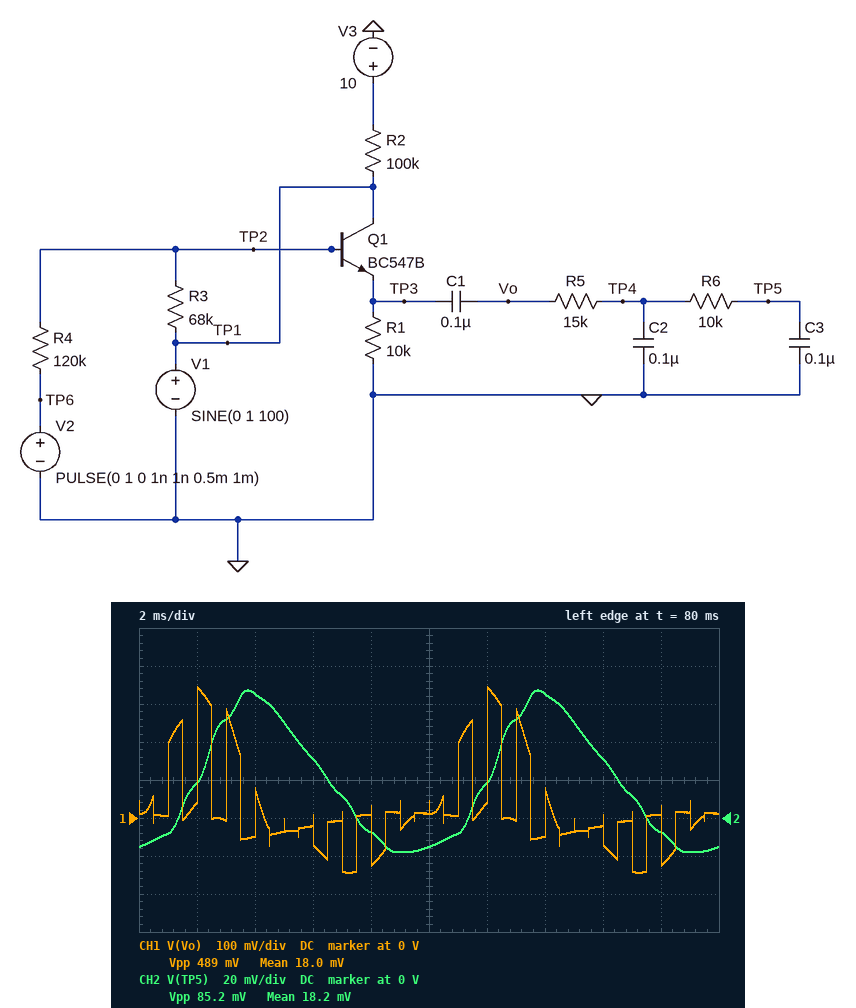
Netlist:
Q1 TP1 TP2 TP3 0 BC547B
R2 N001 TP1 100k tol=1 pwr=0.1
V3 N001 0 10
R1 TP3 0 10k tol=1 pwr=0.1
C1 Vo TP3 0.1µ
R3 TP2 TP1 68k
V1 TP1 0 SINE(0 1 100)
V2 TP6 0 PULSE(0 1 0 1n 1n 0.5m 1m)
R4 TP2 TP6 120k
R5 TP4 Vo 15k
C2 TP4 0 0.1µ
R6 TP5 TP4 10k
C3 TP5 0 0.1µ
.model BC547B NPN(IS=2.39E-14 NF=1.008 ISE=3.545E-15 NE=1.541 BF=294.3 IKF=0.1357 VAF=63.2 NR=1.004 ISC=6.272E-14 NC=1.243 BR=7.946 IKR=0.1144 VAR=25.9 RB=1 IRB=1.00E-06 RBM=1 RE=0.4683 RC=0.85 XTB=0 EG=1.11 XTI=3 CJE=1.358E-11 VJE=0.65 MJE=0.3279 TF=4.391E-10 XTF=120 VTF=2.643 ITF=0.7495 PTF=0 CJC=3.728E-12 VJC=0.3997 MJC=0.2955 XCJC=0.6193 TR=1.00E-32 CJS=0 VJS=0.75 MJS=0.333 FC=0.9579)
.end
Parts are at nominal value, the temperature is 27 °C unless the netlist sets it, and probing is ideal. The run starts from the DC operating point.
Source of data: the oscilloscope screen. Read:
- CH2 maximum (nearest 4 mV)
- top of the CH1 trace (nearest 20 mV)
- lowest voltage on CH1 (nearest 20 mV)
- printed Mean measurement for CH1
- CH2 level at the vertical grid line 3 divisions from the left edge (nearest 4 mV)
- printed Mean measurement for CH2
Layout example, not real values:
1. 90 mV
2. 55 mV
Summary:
1. 68 mV
2. 340 mV
3. -140 mV
4. 18.0 mV
5. 32 mV
6. 18.2 mV
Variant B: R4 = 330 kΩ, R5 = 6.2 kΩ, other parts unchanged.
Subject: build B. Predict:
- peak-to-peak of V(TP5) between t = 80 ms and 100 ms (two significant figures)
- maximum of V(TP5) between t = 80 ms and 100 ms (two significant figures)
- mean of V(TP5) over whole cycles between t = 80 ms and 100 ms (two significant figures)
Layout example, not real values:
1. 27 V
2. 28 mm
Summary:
1. 96 mV
2. 97 mV
3. 31 mV
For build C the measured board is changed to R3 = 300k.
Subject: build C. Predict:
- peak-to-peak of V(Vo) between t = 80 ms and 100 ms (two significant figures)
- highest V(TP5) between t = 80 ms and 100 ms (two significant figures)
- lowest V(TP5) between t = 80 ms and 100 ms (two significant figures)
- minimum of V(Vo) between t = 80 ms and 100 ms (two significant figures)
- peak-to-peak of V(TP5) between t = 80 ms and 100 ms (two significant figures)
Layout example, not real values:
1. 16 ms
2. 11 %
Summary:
1. 690 mV
2. 66 mV
3. -73 mV
4. -330 mV
5. 140 mV
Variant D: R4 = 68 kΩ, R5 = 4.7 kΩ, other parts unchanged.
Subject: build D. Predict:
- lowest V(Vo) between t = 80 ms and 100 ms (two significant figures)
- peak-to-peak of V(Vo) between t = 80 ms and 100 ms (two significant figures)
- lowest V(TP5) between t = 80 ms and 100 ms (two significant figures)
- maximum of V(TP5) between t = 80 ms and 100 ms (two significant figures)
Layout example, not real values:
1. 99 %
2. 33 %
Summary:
1. -280 mV
2. 590 mV
3. -100 mV
4. 92 mV
